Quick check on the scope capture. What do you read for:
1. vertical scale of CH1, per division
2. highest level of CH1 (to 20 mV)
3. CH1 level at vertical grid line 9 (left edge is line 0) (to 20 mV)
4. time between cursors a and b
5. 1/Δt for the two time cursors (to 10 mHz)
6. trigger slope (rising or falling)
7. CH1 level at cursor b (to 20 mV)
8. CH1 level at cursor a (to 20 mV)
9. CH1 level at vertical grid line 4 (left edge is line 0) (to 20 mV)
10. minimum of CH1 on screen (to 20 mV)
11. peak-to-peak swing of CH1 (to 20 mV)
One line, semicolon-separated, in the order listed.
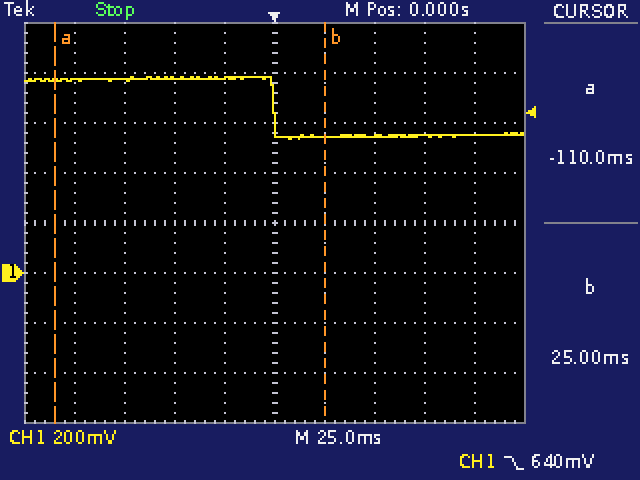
200 mV; 780 mV; 560 mV; 135.0 ms; 7.41 Hz; falling; 540 mV; 780 mV; 780 mV; 540 mV; 240 mV
